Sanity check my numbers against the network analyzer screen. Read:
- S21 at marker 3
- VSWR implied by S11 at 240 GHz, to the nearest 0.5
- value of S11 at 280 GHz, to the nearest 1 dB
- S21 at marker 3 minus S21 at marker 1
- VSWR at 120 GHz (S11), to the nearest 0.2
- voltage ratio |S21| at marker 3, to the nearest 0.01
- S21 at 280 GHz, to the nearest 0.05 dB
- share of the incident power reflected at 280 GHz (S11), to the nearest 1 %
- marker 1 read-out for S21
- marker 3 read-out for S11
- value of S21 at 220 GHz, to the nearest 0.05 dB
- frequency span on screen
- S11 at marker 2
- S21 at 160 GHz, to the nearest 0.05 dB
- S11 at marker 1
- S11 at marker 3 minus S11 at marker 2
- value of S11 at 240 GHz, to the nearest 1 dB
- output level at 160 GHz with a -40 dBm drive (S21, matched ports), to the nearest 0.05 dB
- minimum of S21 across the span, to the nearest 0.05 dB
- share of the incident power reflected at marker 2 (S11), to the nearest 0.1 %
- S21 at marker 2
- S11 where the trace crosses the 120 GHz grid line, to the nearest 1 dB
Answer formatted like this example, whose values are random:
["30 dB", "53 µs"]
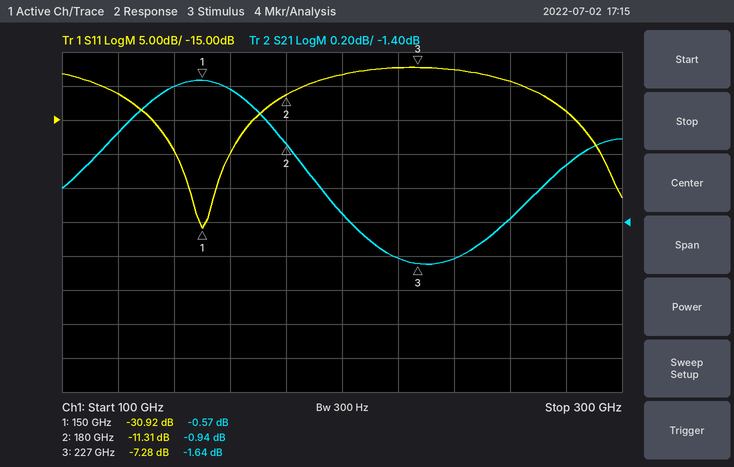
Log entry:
["-1.64 dB", "2.5", "-14 dB", "-1.07 dB", "1.8", "0.83", "-1.05 dB", "4 %", "-0.57 dB", "-7.28 dB", "-1.60 dB", "200 GHz", "-11.31 dB", "-0.60 dB", "-30.92 dB", "4.03 dB", "-8 dB", "-40.60 dBm", "-1.65 dB", "7.4 %", "-0.94 dB", "-11 dB"]
